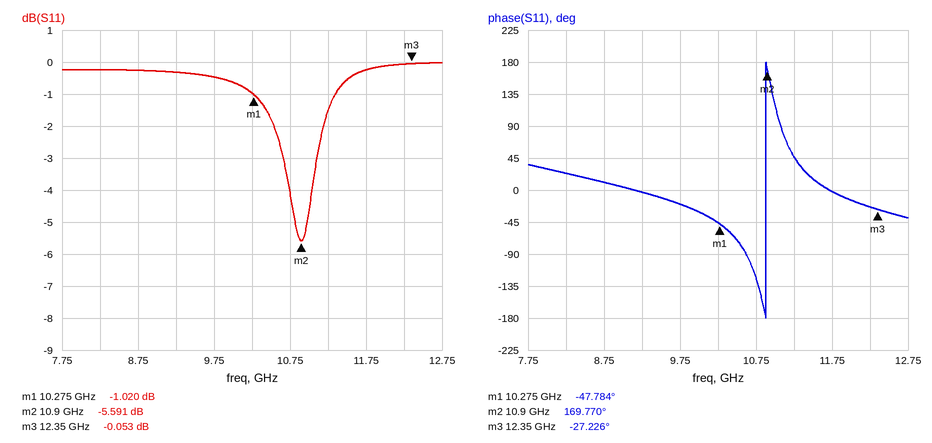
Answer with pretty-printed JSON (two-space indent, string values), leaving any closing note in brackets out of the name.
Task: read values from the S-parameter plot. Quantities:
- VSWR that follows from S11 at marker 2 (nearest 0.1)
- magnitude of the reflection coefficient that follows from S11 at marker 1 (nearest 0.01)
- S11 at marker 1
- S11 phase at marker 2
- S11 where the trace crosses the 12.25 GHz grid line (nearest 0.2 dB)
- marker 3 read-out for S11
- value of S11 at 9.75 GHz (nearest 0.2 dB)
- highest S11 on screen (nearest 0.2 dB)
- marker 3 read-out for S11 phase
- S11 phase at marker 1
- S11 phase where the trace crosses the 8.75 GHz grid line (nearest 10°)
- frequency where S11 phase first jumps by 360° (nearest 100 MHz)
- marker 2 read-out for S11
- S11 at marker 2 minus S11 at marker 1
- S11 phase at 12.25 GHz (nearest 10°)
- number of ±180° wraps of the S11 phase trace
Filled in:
{
  "VSWR that follows from S11 at marker 2": "3.2",
  "magnitude of the reflection coefficient that follows from S11 at marker 1": "0.89",
  "S11 at marker 1": "-1.020 dB",
  "S11 phase at marker 2": "169.770°",
  "S11 where the trace crosses the 12.25 GHz grid line": "0.0 dB",
  "marker 3 read-out for S11": "-0.053 dB",
  "value of S11 at 9.75 GHz": "-0.4 dB",
  "highest S11 on screen": "0.0 dB",
  "marker 3 read-out for S11 phase": "-27.226°",
  "S11 phase at marker 1": "-47.784°",
  "S11 phase where the trace crosses the 8.75 GHz grid line": "10°",
  "frequency where S11 phase first jumps by 360°": "10.9 GHz",
  "marker 2 read-out for S11": "-5.591 dB",
  "S11 at marker 2 minus S11 at marker 1": "-4.571 dB",
  "S11 phase at 12.25 GHz": "-20°",
  "number of ±180° wraps of the S11 phase trace": "1"
}
